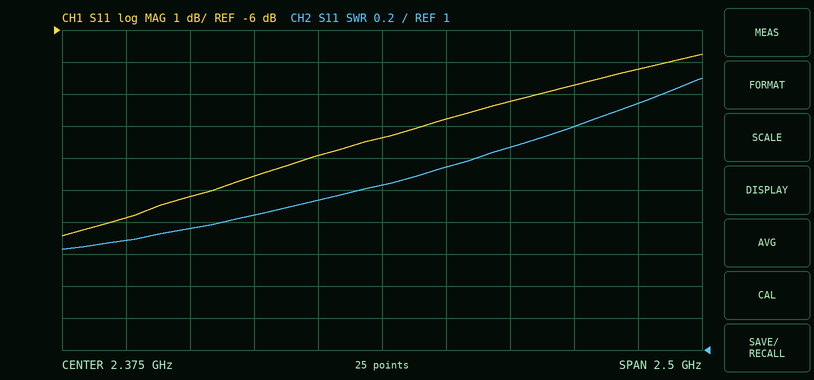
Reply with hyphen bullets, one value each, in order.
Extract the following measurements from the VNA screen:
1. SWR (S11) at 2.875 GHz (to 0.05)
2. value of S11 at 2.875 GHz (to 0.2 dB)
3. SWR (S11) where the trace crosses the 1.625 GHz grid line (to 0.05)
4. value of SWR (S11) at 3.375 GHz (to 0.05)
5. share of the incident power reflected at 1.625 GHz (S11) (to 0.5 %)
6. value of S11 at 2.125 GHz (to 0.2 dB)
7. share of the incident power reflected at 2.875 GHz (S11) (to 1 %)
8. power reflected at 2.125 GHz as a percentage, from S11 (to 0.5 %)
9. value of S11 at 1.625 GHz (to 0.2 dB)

- 2.25
- -8.2 dB
- 1.75
- 2.55
- 7.5 %
- -10.0 dB
- 15 %
- 10.0 %
- -11.2 dB
